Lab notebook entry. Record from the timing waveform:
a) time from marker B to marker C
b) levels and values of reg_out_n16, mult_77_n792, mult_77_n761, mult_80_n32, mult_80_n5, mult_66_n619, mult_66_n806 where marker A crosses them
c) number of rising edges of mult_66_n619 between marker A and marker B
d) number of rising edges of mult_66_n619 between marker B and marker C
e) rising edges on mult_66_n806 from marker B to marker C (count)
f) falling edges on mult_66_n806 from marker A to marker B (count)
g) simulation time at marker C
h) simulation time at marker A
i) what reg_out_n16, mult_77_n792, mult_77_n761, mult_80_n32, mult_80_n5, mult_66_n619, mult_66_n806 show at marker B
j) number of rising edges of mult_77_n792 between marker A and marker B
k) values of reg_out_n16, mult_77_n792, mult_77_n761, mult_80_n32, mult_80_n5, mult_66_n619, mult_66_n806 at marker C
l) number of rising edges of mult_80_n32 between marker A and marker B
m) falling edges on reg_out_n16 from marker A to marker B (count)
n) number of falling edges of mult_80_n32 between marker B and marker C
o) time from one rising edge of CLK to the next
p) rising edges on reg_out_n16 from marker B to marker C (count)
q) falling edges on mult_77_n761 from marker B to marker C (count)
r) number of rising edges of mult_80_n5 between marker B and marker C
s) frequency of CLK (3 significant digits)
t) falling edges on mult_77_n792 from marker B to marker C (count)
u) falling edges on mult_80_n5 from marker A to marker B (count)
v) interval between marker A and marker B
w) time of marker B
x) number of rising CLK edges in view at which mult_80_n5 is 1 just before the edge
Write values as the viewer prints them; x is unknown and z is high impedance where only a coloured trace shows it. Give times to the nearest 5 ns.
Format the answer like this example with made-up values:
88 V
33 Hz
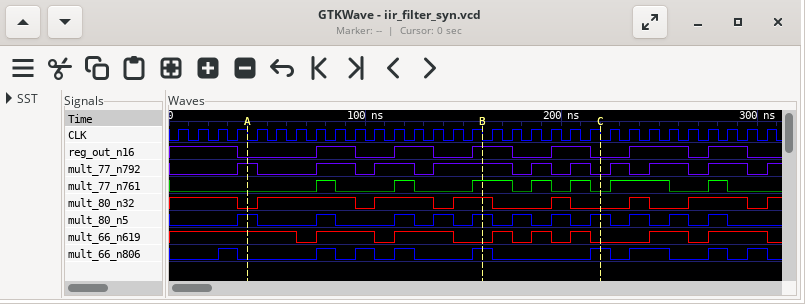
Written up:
60 ns
reg_out_n16=0, mult_77_n792=1, mult_77_n761=0, mult_80_n32=0, mult_80_n5=1, mult_66_n619=1, mult_66_n806=0
2
3
1
3
220 ns
40 ns
reg_out_n16=1, mult_77_n792=1, mult_77_n761=1, mult_80_n32=1, mult_80_n5=1, mult_66_n619=0, mult_66_n806=1
3
reg_out_n16=0, mult_77_n792=0, mult_77_n761=0, mult_80_n32=0, mult_80_n5=1, mult_66_n619=0, mult_66_n806=1
3
2
2
10 ns
1
3
3
100 MHz
3
4
120 ns
160 ns
11
